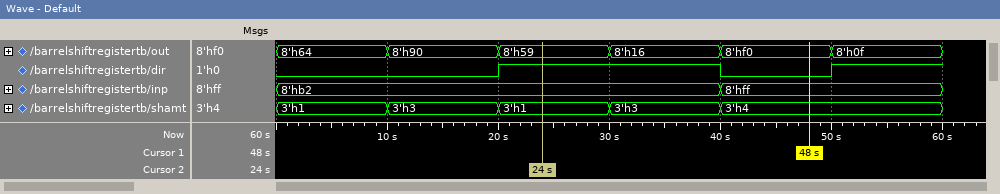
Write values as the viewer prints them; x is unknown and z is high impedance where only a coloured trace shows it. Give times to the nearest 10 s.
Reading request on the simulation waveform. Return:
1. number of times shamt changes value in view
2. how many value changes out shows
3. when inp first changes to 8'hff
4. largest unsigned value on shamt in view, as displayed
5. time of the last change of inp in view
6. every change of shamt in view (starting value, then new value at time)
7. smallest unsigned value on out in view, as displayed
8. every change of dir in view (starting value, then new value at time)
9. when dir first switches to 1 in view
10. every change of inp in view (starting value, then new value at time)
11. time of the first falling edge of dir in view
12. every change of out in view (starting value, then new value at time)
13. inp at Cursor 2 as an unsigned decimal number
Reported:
4
5
40 s
3'h4
40 s
3'h1, 3'h3 at 10 s, 3'h1 at 20 s, 3'h3 at 30 s, 3'h4 at 40 s
8'h0f
0, 1 at 20 s, 0 at 40 s, 1 at 50 s
20 s
8'hb2, 8'hff at 40 s
40 s
8'h64, 8'h90 at 10 s, 8'h59 at 20 s, 8'h16 at 30 s, 8'hf0 at 40 s, 8'h0f at 50 s
178
